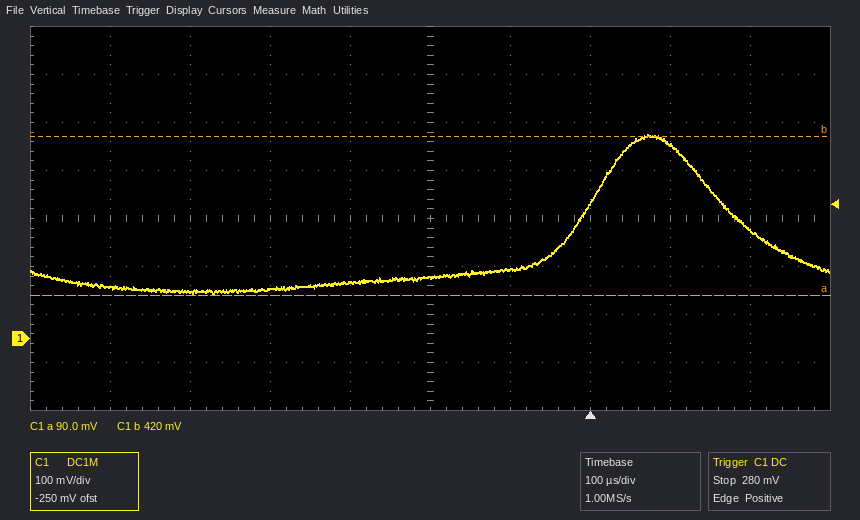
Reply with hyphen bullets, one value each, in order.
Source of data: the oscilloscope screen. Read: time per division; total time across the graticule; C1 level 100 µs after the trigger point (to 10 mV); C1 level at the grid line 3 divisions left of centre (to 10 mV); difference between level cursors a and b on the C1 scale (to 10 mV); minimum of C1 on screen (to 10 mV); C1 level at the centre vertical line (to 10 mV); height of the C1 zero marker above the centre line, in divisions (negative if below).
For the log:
- 100 µs
- 1 ms
- 400 mV
- 100 mV
- 330 mV
- 90 mV
- 130 mV
- -2.5 div
